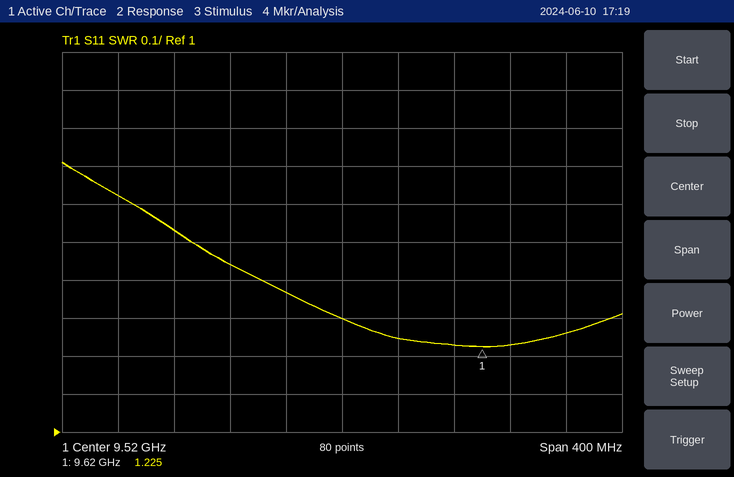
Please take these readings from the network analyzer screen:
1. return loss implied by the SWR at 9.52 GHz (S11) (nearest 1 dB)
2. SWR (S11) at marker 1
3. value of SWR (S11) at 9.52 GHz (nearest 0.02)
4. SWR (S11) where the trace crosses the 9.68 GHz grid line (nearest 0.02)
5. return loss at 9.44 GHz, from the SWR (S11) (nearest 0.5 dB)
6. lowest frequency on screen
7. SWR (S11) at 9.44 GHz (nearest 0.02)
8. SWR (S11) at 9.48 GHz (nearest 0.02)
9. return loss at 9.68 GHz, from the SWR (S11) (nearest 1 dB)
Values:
18 dB
1.225
1.30
1.26
15.0 dB
9.32 GHz
1.44
1.36
19 dB
